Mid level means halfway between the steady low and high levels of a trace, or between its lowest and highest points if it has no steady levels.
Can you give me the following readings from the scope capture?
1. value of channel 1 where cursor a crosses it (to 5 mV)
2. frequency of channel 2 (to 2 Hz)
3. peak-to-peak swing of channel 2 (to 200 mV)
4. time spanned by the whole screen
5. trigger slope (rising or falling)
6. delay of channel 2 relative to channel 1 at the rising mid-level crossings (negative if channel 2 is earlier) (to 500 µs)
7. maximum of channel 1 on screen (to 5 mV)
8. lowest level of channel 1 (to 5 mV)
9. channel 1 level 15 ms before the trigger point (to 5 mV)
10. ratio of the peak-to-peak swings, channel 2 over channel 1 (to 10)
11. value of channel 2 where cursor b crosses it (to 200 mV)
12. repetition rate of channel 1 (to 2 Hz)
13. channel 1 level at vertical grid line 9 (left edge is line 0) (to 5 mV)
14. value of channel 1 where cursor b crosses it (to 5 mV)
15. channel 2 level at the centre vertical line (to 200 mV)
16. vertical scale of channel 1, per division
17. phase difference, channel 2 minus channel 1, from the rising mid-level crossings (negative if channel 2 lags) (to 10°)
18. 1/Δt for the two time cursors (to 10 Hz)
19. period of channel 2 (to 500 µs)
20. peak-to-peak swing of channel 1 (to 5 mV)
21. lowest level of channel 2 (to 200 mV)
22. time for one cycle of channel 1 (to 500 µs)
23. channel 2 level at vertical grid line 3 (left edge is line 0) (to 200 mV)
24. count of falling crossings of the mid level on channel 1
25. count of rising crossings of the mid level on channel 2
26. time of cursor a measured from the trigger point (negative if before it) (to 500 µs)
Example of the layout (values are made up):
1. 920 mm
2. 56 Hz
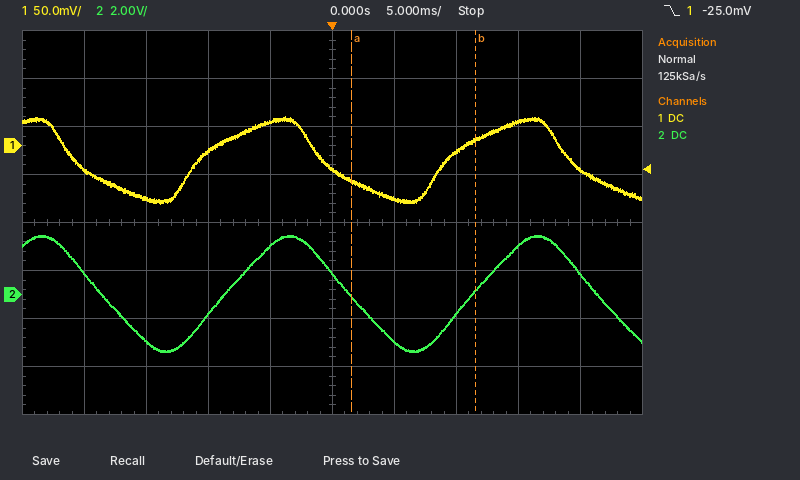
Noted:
1. -35 mV
2. 50 Hz
3. 4.8 V
4. 50 ms
5. falling
6. +2.0 ms
7. 30 mV
8. -60 mV
9. -55 mV
10. 50
11. 200 mV
12. 50 Hz
13. -25 mV
14. 5 mV
15. 800 mV
16. 50 mV
17. -40°
18. 100 Hz
19. 20.0 ms
20. 90 mV
21. -2.4 V
22. 20.0 ms
23. -800 mV
24. 3
25. 2
26. +1.5 ms
